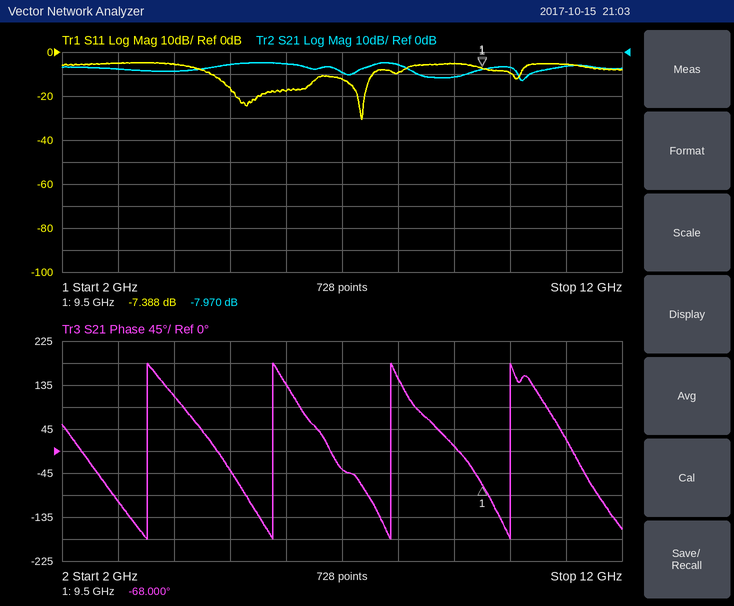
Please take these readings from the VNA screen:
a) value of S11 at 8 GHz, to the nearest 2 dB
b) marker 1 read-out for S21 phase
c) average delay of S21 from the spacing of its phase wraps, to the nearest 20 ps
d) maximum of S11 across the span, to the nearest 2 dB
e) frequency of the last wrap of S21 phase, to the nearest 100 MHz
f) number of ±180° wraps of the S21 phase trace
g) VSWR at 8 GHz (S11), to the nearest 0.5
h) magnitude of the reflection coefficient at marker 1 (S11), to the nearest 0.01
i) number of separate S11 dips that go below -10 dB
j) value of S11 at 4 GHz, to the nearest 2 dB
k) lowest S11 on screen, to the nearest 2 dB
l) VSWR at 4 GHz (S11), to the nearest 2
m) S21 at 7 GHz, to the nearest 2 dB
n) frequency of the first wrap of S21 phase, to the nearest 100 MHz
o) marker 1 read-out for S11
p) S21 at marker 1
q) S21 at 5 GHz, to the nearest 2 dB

-10 dB
-68.000°
460 ps
-4 dB
10.0 GHz
4
2.0
0.43
3
-6 dB
-30 dB
4
-10 dB
3.5 GHz
-7.388 dB
-7.970 dB
-6 dB
